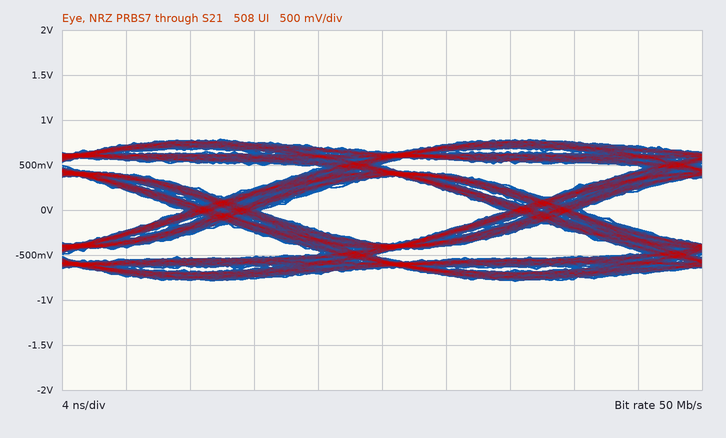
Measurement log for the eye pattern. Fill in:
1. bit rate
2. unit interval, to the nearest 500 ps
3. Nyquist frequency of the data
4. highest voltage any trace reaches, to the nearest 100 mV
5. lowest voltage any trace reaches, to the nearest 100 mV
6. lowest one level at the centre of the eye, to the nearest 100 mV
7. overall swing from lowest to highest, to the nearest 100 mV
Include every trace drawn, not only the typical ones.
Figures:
50 Mb/s
20.0 ns
25 MHz
800 mV
-800 mV
400 mV
1.6 V
